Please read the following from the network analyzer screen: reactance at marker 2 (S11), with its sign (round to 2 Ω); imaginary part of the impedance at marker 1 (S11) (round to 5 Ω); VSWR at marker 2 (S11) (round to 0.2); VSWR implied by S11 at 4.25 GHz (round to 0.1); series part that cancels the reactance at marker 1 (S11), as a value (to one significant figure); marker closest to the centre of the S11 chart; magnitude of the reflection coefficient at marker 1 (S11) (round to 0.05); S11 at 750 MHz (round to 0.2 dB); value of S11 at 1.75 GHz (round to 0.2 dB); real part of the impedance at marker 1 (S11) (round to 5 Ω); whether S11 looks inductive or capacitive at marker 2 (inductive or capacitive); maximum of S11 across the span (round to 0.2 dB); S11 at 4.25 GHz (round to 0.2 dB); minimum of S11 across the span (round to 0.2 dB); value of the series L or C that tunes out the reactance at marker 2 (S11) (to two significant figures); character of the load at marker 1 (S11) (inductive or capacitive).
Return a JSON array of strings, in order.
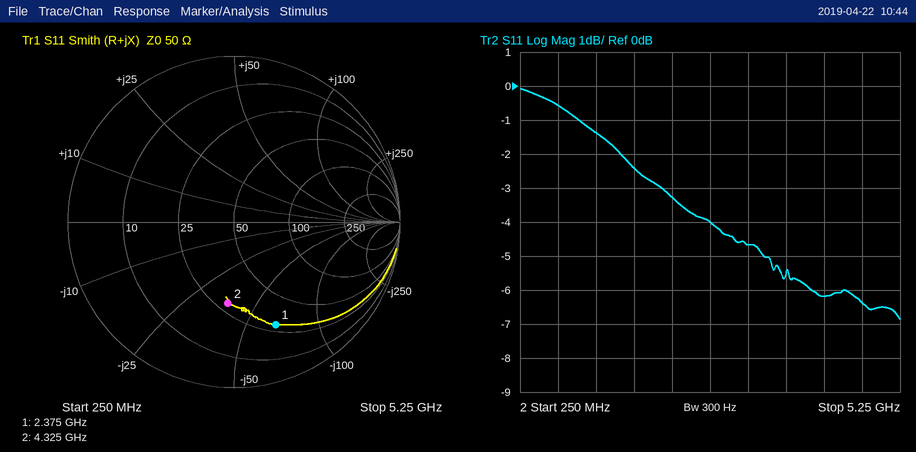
["-38 Ω", "-65 Ω", "3.0", "2.9", "4 nH", "marker 2", "0.65", "-0.6 dB", "-2.4 dB", "30 Ω", "capacitive", "0.0 dB", "-6.2 dB", "-6.8 dB", "1.4 nH", "capacitive"]
